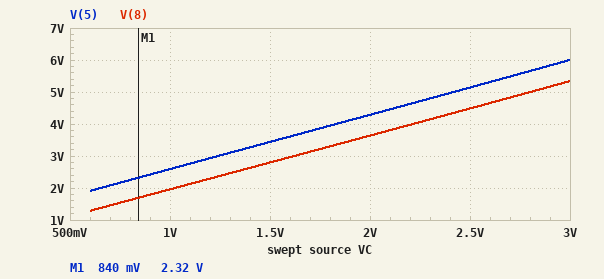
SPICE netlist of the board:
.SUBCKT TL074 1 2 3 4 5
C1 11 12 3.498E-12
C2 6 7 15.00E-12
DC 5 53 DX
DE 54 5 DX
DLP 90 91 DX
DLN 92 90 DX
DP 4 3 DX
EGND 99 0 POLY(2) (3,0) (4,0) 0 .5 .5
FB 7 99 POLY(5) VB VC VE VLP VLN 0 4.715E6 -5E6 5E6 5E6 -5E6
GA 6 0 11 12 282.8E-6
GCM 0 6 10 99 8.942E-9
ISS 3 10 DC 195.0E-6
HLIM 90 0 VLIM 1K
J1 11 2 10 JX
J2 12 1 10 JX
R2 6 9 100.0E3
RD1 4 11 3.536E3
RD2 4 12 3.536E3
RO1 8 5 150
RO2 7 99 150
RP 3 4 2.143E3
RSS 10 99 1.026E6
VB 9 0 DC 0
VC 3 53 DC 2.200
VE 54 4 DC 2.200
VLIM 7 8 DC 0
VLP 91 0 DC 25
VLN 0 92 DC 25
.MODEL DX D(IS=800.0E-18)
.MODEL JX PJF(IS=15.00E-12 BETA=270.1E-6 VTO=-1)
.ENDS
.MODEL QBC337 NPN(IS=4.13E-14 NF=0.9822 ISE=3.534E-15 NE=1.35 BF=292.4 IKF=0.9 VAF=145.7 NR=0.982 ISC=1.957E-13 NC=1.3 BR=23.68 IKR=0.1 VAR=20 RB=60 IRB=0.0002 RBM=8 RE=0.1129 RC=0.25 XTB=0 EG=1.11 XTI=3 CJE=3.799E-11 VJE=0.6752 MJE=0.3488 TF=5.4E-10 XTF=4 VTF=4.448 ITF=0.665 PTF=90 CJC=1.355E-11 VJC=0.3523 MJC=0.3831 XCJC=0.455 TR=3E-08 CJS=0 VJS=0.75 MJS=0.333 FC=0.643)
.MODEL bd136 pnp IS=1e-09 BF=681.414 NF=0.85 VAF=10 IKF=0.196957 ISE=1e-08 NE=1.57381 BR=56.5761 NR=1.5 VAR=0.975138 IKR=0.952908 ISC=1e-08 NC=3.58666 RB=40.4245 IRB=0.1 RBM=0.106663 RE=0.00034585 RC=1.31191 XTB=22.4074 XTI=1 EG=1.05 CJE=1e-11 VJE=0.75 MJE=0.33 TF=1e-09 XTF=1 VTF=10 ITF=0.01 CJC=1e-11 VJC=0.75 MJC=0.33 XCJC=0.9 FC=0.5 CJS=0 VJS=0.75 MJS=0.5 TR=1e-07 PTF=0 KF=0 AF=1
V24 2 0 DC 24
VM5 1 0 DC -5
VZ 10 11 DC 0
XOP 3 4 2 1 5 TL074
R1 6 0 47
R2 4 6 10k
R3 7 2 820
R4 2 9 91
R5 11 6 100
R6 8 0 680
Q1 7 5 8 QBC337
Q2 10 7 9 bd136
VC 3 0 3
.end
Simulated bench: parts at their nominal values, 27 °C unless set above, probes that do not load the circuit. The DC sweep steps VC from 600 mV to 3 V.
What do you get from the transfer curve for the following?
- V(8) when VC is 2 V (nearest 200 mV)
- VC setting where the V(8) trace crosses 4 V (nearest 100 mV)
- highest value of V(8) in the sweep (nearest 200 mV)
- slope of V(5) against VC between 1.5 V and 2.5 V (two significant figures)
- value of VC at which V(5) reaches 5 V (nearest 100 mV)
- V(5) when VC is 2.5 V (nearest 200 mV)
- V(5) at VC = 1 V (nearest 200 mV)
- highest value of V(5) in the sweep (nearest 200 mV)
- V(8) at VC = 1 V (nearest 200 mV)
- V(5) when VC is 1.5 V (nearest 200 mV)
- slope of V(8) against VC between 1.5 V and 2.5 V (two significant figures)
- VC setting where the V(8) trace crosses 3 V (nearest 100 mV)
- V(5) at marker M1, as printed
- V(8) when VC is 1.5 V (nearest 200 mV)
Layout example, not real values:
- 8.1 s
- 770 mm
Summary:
- 3.6 V
- 2.2 V
- 5.4 V
- 1.7 V/V
- 2.4 V
- 5.2 V
- 2.6 V
- 6.0 V
- 2.0 V
- 3.4 V
- 1.7 V/V
- 1.6 V
- 2.32 V
- 2.8 V
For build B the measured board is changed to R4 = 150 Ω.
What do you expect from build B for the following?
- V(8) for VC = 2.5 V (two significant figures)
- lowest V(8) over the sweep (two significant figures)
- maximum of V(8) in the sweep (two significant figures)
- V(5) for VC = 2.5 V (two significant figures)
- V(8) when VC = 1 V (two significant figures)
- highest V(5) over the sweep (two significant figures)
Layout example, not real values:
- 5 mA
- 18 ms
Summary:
- 7.1 V
- 1.9 V
- 8.6 V
- 7.8 V
- 3.0 V
- 9.2 V
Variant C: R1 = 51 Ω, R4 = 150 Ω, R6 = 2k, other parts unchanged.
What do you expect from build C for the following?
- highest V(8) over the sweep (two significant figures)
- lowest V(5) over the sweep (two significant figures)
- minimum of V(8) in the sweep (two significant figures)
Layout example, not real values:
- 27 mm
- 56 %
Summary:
- 22 V
- 5.9 V
- 5.3 V
